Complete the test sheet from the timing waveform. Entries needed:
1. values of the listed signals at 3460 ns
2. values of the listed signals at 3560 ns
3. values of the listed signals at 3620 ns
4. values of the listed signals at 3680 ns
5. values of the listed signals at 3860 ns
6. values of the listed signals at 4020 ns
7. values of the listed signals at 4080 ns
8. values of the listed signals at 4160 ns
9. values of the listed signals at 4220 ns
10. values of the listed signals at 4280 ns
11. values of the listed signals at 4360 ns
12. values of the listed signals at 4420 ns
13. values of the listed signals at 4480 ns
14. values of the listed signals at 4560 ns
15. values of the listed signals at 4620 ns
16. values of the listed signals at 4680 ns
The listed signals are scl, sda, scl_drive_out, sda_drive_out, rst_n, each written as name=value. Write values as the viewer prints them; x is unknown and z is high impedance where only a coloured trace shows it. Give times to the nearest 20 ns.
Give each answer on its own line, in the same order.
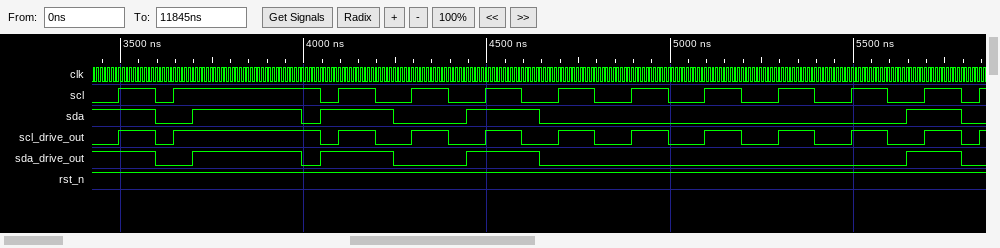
scl=0, sda=1, scl_drive_out=0, sda_drive_out=1, rst_n=1
scl=1, sda=1, scl_drive_out=1, sda_drive_out=1, rst_n=1
scl=0, sda=0, scl_drive_out=0, sda_drive_out=0, rst_n=1
scl=1, sda=0, scl_drive_out=1, sda_drive_out=0, rst_n=1
scl=1, sda=1, scl_drive_out=1, sda_drive_out=1, rst_n=1
scl=1, sda=0, scl_drive_out=1, sda_drive_out=0, rst_n=1
scl=0, sda=1, scl_drive_out=0, sda_drive_out=1, rst_n=1
scl=1, sda=1, scl_drive_out=1, sda_drive_out=1, rst_n=1
scl=0, sda=1, scl_drive_out=0, sda_drive_out=1, rst_n=1
scl=0, sda=0, scl_drive_out=0, sda_drive_out=0, rst_n=1
scl=1, sda=0, scl_drive_out=1, sda_drive_out=0, rst_n=1
scl=0, sda=0, scl_drive_out=0, sda_drive_out=0, rst_n=1
scl=0, sda=1, scl_drive_out=0, sda_drive_out=1, rst_n=1
scl=1, sda=1, scl_drive_out=1, sda_drive_out=1, rst_n=1
scl=0, sda=1, scl_drive_out=0, sda_drive_out=1, rst_n=1
scl=0, sda=0, scl_drive_out=0, sda_drive_out=0, rst_n=1
